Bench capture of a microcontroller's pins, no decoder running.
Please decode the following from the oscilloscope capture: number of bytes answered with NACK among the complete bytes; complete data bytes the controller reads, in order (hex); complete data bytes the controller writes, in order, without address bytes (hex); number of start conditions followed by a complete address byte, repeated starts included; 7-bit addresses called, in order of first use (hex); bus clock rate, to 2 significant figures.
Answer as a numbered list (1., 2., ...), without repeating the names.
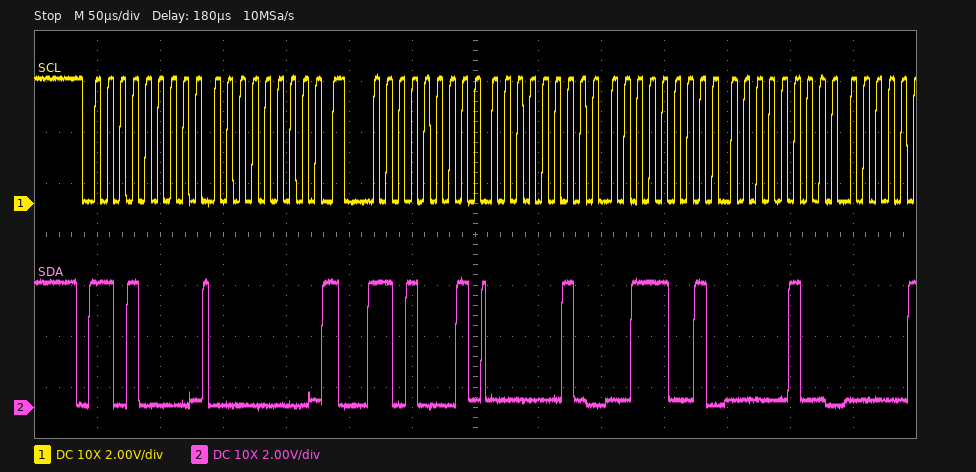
1. 0
2. 02 39 04
3. 00
4. 2
5. 0x68
6. 100 kHz
